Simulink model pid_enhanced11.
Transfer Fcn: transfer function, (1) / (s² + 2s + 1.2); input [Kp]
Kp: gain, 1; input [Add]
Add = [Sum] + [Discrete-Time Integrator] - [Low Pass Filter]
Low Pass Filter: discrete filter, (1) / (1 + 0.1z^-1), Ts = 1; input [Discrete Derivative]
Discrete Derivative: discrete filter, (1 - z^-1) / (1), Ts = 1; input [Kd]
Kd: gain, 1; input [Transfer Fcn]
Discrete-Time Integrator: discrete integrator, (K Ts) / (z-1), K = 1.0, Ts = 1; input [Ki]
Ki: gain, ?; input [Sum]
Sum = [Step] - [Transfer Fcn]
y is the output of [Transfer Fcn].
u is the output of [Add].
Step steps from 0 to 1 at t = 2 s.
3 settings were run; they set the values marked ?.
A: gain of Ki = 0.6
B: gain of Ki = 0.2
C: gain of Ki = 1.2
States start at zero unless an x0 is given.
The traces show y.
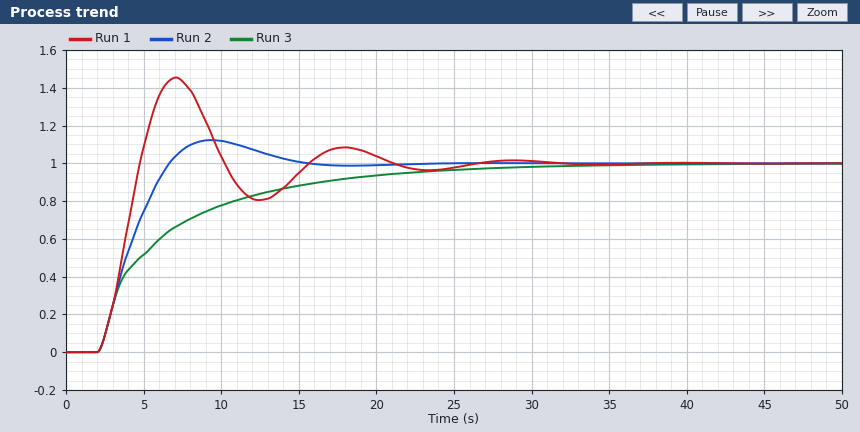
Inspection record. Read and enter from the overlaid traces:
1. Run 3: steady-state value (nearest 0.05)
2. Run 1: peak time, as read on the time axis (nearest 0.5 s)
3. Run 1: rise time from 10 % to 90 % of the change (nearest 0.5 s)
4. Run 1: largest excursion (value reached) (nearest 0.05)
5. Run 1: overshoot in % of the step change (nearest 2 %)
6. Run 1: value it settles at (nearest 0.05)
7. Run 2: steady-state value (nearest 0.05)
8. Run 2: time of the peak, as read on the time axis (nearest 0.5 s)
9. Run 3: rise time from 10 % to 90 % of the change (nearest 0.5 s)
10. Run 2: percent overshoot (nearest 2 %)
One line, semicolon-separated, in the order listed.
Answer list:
1.00; 7.0 s; 2.0 s; 1.45; 46 %; 1.00; 1.00; 9.5 s; 14.0 s; 12 %
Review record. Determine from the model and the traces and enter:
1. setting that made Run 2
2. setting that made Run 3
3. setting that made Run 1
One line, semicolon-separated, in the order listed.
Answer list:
A; B; C
